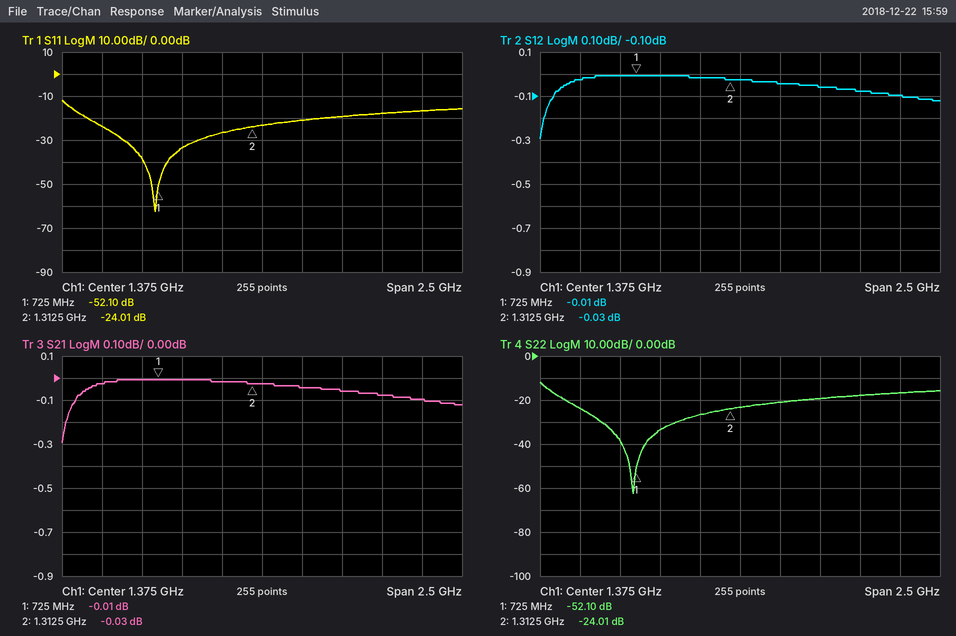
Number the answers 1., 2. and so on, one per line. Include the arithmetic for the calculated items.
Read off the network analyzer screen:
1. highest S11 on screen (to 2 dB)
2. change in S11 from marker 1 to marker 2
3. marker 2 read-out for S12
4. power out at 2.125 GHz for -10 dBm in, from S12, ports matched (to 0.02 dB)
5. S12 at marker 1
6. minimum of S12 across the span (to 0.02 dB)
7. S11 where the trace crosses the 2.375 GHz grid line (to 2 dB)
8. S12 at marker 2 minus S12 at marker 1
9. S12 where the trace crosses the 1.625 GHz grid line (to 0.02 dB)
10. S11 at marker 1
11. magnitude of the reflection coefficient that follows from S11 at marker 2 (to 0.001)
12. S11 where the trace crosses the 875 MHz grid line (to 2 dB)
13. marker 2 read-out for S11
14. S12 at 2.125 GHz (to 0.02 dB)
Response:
1. -12 dB
2. -24.01 − (-52.1) = 28.09 dB
3. -0.03 dB
4. -10 dBm + (-0.08 dB) = -10.08 dBm
5. -0.01 dB
6. -0.30 dB
7. -16 dB
8. -0.03 − (-0.01) = -0.02 dB
9. -0.04 dB
10. -52.10 dB
11. 10^(-24.01/20) ≈ 0.063
12. -34 dB
13. -24.01 dB
14. -0.08 dB
